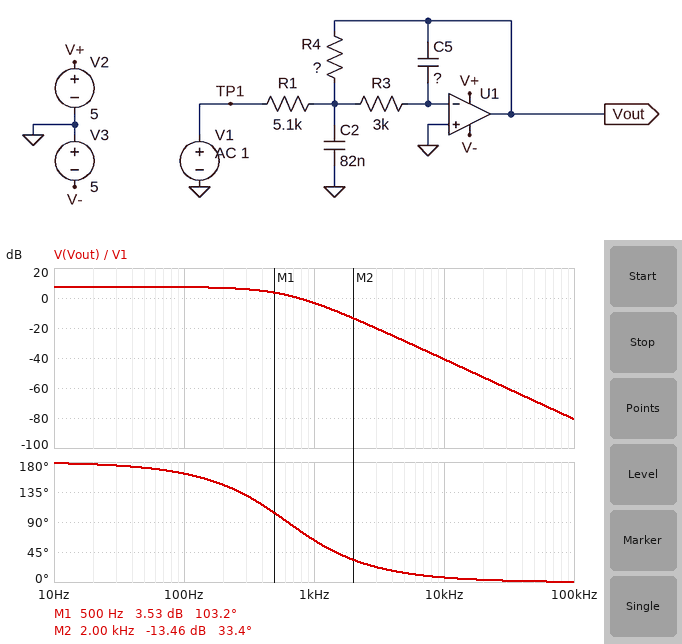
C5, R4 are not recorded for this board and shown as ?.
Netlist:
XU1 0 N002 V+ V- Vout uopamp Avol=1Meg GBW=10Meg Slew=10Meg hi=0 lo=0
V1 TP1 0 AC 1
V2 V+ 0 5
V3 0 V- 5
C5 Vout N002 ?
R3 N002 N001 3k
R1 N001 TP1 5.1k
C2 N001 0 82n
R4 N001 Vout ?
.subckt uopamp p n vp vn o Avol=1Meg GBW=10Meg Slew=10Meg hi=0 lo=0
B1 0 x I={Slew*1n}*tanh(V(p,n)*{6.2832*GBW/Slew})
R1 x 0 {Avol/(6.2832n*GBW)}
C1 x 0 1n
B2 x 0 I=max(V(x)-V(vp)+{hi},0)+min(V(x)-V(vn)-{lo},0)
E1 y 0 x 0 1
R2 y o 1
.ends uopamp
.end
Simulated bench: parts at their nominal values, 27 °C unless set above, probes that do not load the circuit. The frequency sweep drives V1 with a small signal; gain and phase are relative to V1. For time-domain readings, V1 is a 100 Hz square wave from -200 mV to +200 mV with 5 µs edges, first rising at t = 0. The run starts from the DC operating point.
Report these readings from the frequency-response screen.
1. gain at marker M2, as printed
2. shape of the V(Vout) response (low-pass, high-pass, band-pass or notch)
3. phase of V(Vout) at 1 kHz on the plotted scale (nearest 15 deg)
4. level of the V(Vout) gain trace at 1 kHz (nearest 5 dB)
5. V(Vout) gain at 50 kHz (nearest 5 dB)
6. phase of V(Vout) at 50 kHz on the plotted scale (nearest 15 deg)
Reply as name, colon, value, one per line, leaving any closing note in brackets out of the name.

gain at marker M2, as printed: -13.46 dB
shape of the V(Vout) response: low-pass
phase of V(Vout) at 1 kHz on the plotted scale: 60 deg
level of the V(Vout) gain trace at 1 kHz: -5 dB
V(Vout) gain at 50 kHz: -70 dB
phase of V(Vout) at 50 kHz on the plotted scale: 0 deg
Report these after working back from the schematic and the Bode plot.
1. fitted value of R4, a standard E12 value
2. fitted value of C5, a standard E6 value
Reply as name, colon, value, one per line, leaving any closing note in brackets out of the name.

fitted value of R4, a standard E12 value: 12 kΩ
fitted value of C5, a standard E6 value: 22 nF
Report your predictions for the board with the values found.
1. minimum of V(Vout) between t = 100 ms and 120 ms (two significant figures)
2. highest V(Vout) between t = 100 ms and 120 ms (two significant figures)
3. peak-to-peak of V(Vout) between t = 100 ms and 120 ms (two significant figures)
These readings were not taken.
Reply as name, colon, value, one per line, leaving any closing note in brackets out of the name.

minimum of V(Vout) between t = 100 ms and 120 ms: -470 mV
highest V(Vout) between t = 100 ms and 120 ms: 470 mV
peak-to-peak of V(Vout) between t = 100 ms and 120 ms: 940 mV
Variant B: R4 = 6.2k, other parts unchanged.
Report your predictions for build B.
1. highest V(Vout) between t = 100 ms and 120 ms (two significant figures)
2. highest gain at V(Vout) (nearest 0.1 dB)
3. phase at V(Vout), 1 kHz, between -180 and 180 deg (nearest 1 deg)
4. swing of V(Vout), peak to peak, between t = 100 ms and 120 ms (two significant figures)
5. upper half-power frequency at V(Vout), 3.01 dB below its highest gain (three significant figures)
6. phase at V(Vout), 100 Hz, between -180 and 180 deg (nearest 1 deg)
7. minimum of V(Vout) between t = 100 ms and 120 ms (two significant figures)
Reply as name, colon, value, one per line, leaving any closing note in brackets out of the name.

highest V(Vout) between t = 100 ms and 120 ms: 250 mV
highest gain at V(Vout): 1.7 dB
phase at V(Vout), 1 kHz, between -180 and 180 deg: 80 deg
swing of V(Vout), peak to peak, between t = 100 ms and 120 ms: 510 mV
upper half-power frequency at V(Vout), 3.01 dB below its highest gain: 790 Hz
phase at V(Vout), 100 Hz, between -180 and 180 deg: 170 deg
minimum of V(Vout) between t = 100 ms and 120 ms: -250 mV
